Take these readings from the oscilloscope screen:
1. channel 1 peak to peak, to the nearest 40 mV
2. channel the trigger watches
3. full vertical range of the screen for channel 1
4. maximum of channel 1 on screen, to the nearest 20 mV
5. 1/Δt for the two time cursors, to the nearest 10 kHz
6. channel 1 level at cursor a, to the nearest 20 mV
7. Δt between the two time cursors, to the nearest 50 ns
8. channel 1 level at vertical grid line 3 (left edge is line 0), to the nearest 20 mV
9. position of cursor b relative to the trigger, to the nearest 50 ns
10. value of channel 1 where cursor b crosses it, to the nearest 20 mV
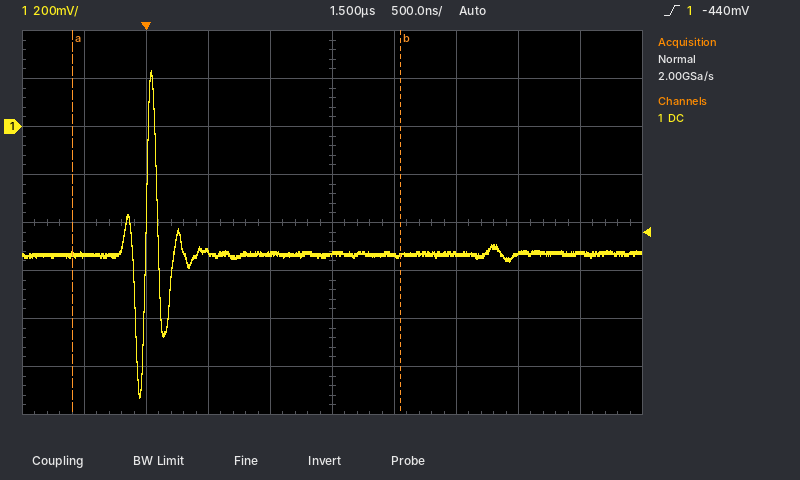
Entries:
1.36 V
channel 1
1.6 V
240 mV
380 kHz
-540 mV
2.65 µs
-520 mV
+2.05 µs
-540 mV
